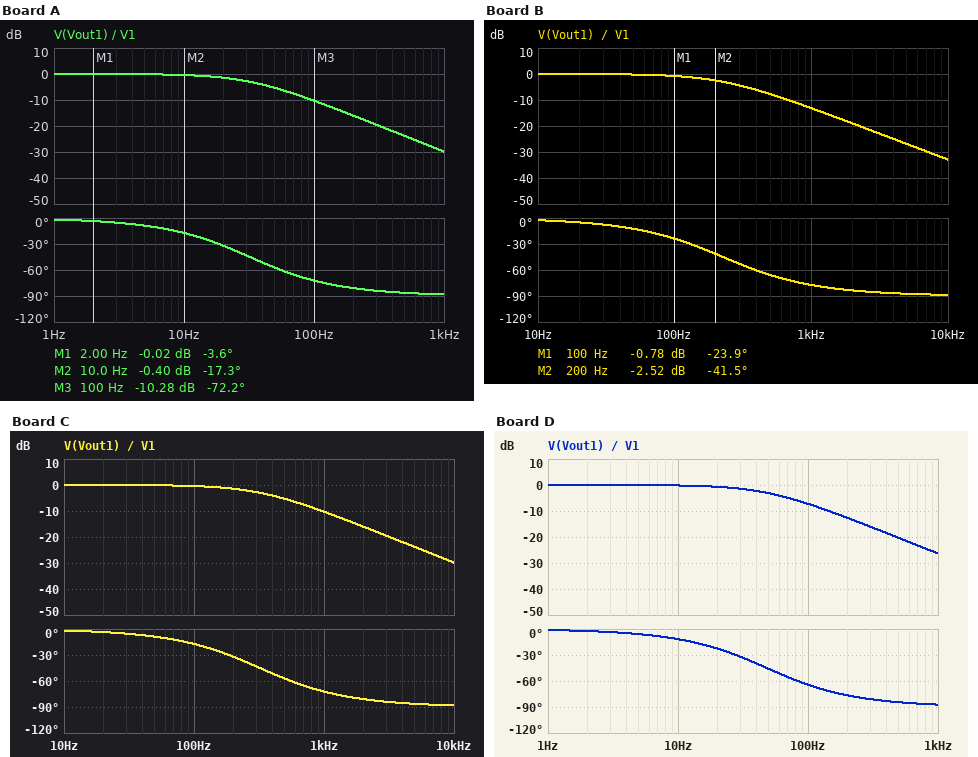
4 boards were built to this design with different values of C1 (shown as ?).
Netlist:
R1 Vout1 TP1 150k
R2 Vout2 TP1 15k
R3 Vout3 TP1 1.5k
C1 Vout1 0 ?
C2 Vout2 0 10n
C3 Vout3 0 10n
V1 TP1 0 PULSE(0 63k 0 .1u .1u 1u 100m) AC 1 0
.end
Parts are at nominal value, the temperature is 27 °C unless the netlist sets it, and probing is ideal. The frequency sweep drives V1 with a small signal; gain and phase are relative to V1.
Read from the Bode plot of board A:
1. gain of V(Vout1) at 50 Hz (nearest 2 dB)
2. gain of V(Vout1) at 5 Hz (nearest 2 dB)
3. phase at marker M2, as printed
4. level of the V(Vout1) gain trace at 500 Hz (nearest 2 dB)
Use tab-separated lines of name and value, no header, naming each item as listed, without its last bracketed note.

gain of V(Vout1) at 50 Hz	-6 dB
gain of V(Vout1) at 5 Hz	0 dB
phase at marker M2, as printed	-17.3 deg
level of the V(Vout1) gain trace at 500 Hz	-24 dB
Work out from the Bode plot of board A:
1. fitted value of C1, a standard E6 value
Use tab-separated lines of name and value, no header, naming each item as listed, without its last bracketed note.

fitted value of C1, a standard E6 value	33 nF
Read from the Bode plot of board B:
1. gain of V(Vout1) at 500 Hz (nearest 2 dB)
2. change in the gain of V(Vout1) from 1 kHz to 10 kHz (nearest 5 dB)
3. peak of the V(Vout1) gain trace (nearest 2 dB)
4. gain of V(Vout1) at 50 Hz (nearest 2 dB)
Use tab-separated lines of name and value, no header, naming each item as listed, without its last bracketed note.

gain of V(Vout1) at 500 Hz	-8 dB
change in the gain of V(Vout1) from 1 kHz to 10 kHz	-20 dB
peak of the V(Vout1) gain trace	0 dB
gain of V(Vout1) at 50 Hz	0 dB
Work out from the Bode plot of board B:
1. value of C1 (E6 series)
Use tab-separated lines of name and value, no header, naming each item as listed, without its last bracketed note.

value of C1	4.7 nF
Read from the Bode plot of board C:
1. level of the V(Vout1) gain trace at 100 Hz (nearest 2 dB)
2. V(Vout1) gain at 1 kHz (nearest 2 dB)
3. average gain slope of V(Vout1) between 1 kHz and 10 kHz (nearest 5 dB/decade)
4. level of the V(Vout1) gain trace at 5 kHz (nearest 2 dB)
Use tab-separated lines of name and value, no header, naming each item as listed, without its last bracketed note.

level of the V(Vout1) gain trace at 100 Hz	0 dB
V(Vout1) gain at 1 kHz	-10 dB
average gain slope of V(Vout1) between 1 kHz and 10 kHz	-20 dB/decade
level of the V(Vout1) gain trace at 5 kHz	-24 dB
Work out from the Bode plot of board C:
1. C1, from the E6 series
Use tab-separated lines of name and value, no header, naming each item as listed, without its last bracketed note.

C1, from the E6 series	3.3 nF
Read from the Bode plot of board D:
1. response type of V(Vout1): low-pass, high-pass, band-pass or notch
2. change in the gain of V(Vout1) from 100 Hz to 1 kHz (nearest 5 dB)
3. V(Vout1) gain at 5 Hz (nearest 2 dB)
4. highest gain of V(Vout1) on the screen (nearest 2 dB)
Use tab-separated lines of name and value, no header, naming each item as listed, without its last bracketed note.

response type of V(Vout1): low-pass, high-pass, band-pass or notch	low-pass
change in the gain of V(Vout1) from 100 Hz to 1 kHz	-20 dB
V(Vout1) gain at 5 Hz	0 dB
highest gain of V(Vout1) on the screen	0 dB
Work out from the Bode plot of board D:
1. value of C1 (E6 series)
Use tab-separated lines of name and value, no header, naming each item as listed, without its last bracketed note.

value of C1	22 nF
